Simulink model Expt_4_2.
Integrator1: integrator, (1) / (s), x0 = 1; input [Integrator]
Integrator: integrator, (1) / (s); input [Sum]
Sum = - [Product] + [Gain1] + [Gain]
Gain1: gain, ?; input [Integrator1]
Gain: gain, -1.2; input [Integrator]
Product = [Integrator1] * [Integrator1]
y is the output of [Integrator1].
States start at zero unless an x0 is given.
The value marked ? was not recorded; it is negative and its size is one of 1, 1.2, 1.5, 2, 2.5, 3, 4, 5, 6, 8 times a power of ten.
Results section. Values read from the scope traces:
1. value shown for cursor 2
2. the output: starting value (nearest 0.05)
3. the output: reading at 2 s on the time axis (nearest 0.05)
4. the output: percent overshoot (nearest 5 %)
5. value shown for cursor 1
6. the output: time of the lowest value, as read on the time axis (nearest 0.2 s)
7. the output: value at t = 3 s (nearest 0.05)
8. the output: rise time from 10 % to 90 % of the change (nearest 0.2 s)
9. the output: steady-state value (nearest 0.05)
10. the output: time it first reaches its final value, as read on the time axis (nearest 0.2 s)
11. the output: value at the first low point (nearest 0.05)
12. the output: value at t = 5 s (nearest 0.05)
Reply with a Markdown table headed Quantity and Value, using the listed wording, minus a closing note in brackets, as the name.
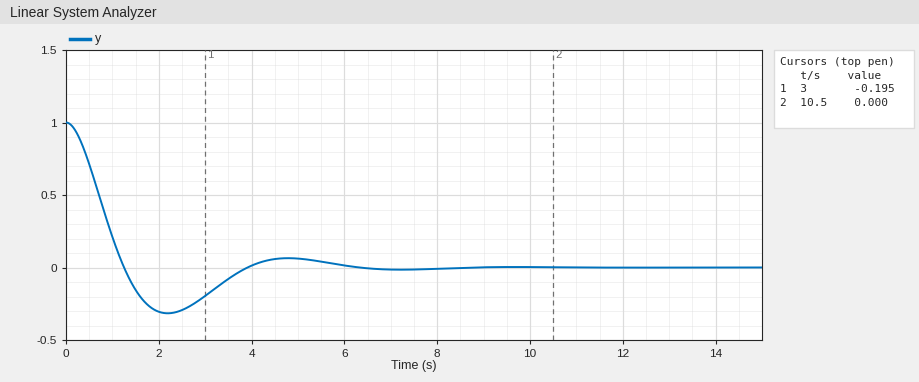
| Quantity | Value |
|---|---|
| value shown for cursor 2 | 0.000 |
| the output: starting value | 1.00 |
| the output: reading at 2 s on the time axis | -0.30 |
| the output: percent overshoot | 30 % |
| value shown for cursor 1 | -0.195 |
| the output: time of the lowest value, as read on the time axis | 2.2 s |
| the output: value at t = 3 s | -0.20 |
| the output: rise time from 10 % to 90 % of the change | 0.8 s |
| the output: steady-state value | 0.00 |
| the output: time it first reaches its final value, as read on the time axis | 1.2 s |
| the output: value at the first low point | -0.30 |
| the output: value at t = 5 s | 0.05 |
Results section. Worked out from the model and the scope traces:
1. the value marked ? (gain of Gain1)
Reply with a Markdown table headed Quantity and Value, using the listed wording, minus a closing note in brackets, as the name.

| Quantity | Value |
|---|---|
| the value marked ? | -2 |
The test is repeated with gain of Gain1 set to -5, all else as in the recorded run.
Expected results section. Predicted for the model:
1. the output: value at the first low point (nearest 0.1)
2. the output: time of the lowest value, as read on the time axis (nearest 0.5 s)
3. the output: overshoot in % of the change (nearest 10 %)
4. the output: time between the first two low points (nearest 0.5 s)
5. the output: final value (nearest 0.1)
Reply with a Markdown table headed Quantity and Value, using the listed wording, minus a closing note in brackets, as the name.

| Quantity | Value |
|---|---|
| the output: value at the first low point | -0.5 |
| the output: time of the lowest value, as read on the time axis | 1.5 s |
| the output: overshoot in % of the change | 50 % |
| the output: time between the first two low points | 3.0 s |
| the output: final value | 0.0 |
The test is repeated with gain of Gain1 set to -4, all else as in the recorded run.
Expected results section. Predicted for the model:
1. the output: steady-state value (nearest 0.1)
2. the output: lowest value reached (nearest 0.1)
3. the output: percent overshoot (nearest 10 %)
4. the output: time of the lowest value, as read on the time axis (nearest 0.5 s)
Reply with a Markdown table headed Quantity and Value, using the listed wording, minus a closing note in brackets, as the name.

| Quantity | Value |
|---|---|
| the output: steady-state value | 0.0 |
| the output: lowest value reached | -0.4 |
| the output: percent overshoot | 40 % |
| the output: time of the lowest value, as read on the time axis | 1.5 s |
